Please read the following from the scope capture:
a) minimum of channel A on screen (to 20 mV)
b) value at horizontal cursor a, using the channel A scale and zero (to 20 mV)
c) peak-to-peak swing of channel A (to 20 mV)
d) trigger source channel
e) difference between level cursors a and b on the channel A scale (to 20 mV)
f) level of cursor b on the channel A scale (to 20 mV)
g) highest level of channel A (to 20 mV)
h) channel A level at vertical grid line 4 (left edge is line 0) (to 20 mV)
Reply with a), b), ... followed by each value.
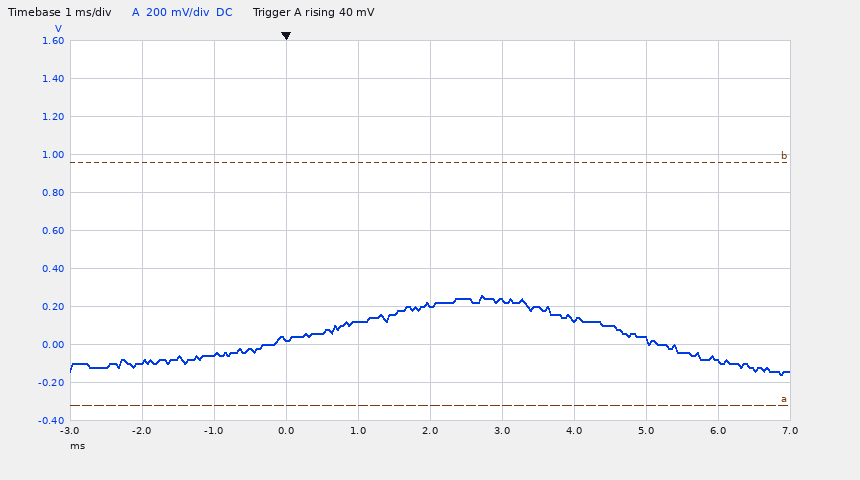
a) -160 mV
b) -320 mV
c) 420 mV
d) channel A
e) 1.28 V
f) 960 mV
g) 260 mV
h) 120 mV
